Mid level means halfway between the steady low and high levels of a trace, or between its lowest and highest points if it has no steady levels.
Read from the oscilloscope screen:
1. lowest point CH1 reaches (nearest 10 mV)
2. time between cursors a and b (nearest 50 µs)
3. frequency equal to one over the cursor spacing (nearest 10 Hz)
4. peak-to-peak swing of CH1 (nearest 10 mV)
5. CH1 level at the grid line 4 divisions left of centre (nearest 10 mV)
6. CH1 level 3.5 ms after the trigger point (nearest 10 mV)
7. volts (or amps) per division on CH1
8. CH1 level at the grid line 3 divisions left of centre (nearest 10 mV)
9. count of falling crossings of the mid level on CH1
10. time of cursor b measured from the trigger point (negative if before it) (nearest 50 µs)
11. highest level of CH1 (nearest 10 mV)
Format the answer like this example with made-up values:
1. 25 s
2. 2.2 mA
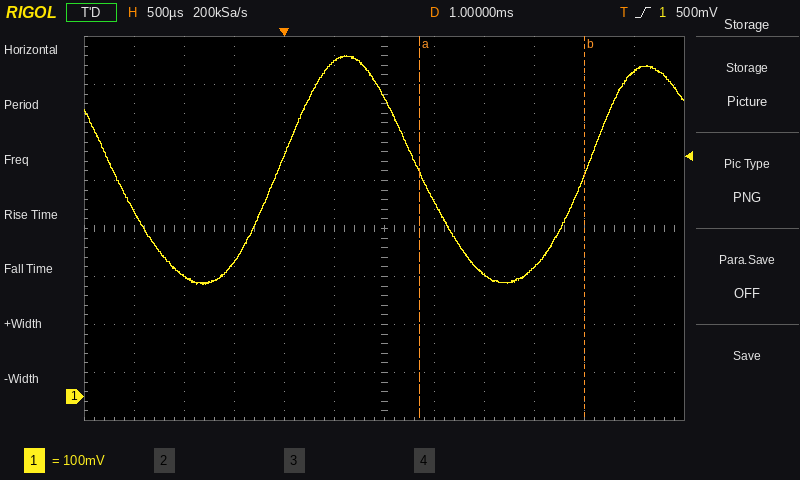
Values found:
1. 230 mV
2. 1.65 ms
3. 610 Hz
4. 480 mV
5. 250 mV
6. 680 mV
7. 100 mV
8. 280 mV
9. 2
10. +3.00 ms
11. 710 mV
